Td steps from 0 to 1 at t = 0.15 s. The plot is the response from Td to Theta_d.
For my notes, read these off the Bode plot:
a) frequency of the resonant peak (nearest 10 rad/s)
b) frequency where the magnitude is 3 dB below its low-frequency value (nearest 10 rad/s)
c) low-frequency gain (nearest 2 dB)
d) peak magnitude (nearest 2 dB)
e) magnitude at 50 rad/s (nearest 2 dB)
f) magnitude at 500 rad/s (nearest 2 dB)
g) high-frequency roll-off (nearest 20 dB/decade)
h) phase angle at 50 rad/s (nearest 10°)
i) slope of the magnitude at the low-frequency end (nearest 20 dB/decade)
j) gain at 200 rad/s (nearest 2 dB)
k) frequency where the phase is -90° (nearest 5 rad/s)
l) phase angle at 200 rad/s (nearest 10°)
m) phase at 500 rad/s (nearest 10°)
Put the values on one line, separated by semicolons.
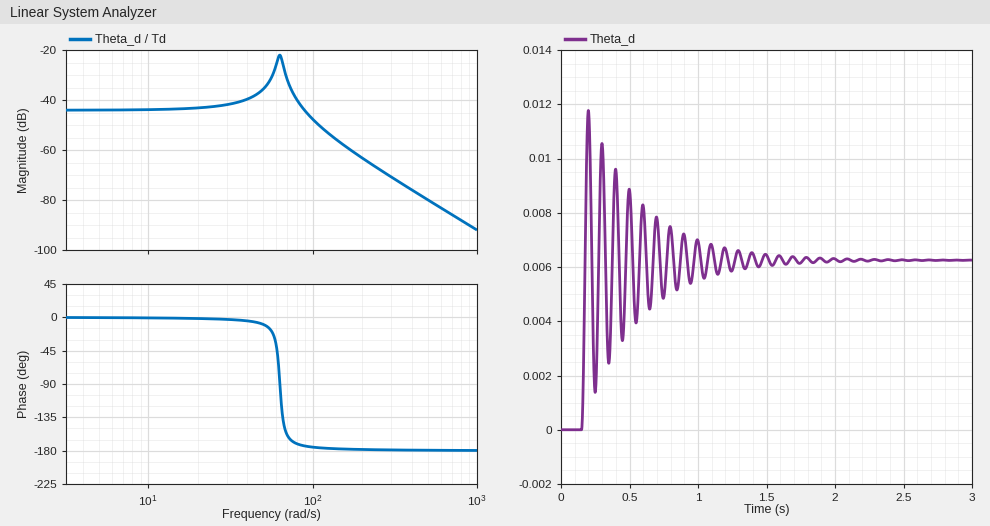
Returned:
60 rad/s; 100 rad/s; -44 dB; -22 dB; -36 dB; -80 dB; -40 dB/decade; -10°; 0 dB/decade; -64 dB; 65 rad/s; -180°; -180°
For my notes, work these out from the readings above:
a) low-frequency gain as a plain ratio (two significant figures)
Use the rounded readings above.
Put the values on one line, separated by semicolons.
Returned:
0.0063
